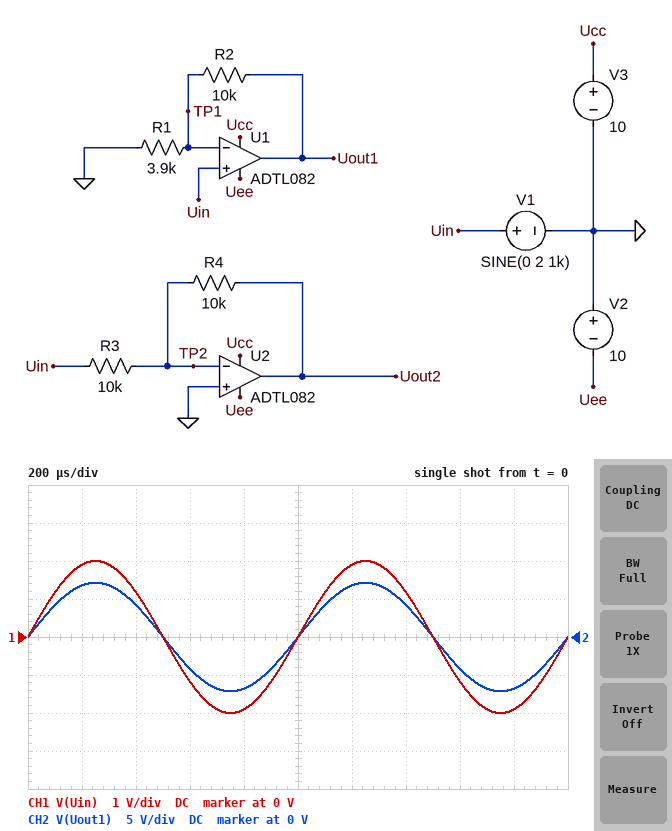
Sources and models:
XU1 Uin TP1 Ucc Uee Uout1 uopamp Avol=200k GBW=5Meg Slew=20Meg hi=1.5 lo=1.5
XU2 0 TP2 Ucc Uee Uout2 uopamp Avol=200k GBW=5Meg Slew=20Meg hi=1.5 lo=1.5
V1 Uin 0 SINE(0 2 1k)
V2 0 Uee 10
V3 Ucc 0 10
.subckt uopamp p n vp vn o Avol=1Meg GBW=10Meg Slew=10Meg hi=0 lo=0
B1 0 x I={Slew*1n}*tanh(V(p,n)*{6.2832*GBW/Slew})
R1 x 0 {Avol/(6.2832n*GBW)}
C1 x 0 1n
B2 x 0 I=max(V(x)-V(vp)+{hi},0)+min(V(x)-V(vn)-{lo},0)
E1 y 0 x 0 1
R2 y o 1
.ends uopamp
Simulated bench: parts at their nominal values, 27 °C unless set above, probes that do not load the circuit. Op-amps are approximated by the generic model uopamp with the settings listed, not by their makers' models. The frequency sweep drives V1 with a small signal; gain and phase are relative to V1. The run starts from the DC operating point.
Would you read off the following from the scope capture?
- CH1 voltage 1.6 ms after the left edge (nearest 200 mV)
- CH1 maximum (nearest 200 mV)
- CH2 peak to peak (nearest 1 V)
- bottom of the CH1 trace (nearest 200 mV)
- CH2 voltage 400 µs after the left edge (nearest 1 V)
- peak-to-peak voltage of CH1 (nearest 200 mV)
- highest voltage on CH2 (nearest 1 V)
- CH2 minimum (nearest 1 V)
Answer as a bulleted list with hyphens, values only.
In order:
- -1.2 V
- 2.0 V
- 14 V
- -2.0 V
- 4 V
- 4.0 V
- 7 V
- -7 V
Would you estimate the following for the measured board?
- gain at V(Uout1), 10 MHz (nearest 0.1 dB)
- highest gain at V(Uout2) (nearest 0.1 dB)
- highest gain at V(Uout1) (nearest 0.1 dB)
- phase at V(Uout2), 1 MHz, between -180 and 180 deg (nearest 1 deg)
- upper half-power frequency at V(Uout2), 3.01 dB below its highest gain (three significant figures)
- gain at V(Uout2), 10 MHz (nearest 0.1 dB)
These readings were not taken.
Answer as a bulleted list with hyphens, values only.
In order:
- -6.1 dB
- 0 dB
- 11.0 dB
- 158 deg
- 2.50 MHz
- -12.3 dB
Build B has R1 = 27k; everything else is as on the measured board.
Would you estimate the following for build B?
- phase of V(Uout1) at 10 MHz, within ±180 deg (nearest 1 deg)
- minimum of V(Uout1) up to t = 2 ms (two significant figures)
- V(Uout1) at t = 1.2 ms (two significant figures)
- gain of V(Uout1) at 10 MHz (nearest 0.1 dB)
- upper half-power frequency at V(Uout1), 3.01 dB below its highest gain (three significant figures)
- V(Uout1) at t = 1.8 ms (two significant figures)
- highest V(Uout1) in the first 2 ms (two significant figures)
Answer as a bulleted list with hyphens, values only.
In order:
- -70 deg
- -2.7 V
- 2.6 V
- -6.6 dB
- 3.65 MHz
- -2.6 V
- 2.7 V
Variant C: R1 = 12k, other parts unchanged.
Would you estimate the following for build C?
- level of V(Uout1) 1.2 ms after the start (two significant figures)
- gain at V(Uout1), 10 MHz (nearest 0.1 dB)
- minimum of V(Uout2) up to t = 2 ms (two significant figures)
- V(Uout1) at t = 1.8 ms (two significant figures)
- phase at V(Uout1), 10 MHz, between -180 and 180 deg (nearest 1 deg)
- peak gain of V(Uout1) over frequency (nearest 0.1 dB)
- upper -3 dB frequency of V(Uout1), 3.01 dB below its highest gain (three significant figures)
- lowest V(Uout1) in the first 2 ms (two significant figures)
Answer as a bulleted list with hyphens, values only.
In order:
- 3.5 V
- -6.3 dB
- -2.0 V
- -3.5 V
- -75 deg
- 5.3 dB
- 2.73 MHz
- -3.7 V
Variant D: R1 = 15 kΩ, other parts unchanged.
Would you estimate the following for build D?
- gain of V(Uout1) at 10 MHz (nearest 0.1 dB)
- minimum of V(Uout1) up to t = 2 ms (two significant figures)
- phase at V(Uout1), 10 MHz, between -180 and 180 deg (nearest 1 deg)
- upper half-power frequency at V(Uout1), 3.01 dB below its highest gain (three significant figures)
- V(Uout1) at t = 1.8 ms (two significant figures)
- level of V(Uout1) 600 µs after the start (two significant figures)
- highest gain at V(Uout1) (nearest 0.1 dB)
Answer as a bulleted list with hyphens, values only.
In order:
- -6.4 dB
- -3.3 V
- -73 deg
- 3.00 MHz
- -3.2 V
- -2.0 V
- 4.4 dB
